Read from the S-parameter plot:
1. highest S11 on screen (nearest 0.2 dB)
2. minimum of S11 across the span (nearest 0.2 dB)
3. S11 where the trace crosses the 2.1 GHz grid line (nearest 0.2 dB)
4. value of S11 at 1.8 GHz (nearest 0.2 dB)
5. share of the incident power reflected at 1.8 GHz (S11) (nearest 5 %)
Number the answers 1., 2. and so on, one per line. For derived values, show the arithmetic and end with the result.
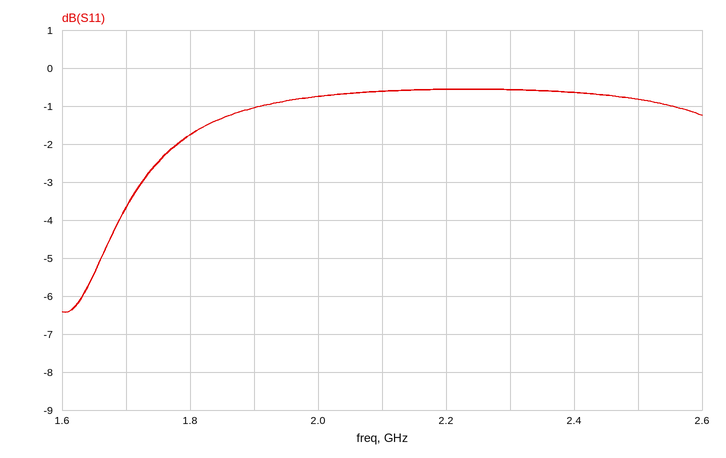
1. -0.6 dB
2. -6.4 dB
3. -0.6 dB
4. -1.8 dB
5. 10^(-1.8/10) ≈ 66.1 %, so 65 % to the nearest 5 %
